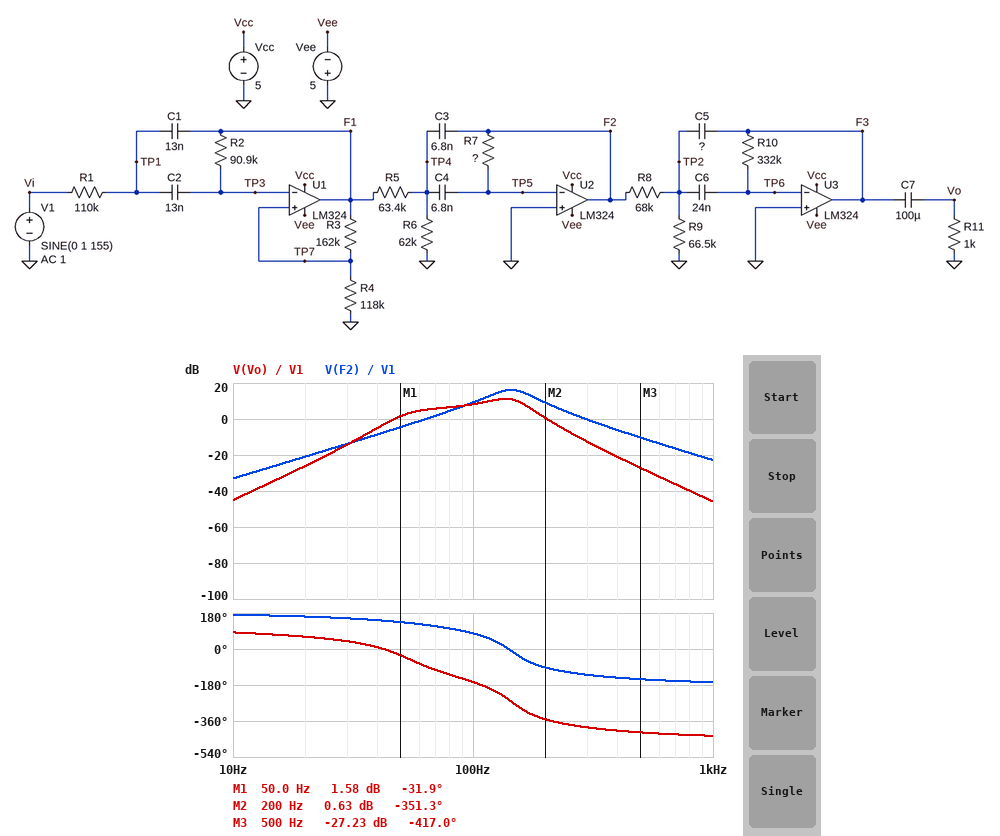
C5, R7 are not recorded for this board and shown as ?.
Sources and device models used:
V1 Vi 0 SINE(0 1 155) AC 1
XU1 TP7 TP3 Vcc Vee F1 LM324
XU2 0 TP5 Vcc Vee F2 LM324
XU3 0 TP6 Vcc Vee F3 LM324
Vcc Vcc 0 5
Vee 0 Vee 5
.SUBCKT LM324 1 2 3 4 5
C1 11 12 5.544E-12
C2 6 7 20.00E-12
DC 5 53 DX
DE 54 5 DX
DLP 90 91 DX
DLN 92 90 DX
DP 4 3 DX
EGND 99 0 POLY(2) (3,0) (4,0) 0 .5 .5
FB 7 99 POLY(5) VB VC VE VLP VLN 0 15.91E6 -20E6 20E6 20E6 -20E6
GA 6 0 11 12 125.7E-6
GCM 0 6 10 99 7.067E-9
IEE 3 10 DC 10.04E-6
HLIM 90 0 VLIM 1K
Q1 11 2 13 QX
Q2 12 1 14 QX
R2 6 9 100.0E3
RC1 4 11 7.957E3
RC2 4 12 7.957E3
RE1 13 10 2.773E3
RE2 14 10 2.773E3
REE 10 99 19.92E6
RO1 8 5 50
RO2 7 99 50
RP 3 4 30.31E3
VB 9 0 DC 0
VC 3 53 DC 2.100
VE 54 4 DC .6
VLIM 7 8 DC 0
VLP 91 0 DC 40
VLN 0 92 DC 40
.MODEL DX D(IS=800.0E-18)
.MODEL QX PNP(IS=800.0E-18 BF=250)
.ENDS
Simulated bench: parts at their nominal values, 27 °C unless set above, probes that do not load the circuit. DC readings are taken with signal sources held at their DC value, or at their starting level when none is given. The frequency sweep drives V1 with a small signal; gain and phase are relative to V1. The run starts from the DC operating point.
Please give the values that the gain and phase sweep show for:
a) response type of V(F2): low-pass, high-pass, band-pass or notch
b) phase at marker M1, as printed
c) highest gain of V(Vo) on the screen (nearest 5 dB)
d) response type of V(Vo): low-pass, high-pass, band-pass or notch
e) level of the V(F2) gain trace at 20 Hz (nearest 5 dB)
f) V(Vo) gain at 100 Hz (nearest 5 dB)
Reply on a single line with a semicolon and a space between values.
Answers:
band-pass; -31.9 deg; 10 dB; band-pass; -20 dB; 10 dB
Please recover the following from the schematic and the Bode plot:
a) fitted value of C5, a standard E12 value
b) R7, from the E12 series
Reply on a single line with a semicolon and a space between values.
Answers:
33 nF; 820 kΩ
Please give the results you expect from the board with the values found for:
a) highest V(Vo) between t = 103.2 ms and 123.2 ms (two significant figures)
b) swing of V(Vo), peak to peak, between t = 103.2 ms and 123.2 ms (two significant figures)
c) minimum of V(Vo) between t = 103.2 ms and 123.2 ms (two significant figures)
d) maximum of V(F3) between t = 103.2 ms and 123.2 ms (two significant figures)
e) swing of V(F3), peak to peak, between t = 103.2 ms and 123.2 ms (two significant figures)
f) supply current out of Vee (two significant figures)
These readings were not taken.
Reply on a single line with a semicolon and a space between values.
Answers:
2.2 V; 4.3 V; -2.1 V; 2.2 V; 4.3 V; 1.0 mA
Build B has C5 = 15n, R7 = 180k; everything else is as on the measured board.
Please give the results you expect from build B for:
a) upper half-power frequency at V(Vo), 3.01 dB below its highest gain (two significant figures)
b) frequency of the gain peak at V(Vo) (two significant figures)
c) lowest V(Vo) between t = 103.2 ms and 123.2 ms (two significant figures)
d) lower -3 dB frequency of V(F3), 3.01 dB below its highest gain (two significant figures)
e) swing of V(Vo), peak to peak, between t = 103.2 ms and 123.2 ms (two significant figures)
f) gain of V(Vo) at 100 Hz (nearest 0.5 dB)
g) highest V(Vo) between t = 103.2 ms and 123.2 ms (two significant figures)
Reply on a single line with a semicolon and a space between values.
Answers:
210 Hz; 99 Hz; -830 mV; 73 Hz; 1.7 V; 0 dB; 830 mV
